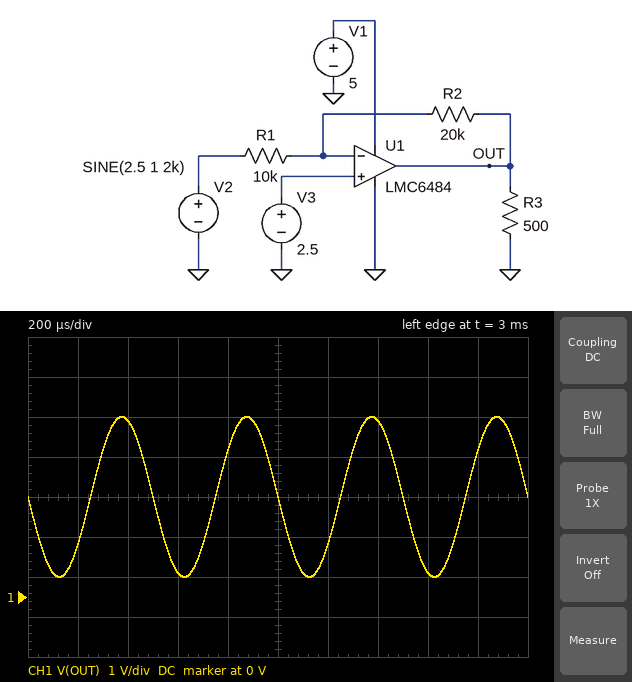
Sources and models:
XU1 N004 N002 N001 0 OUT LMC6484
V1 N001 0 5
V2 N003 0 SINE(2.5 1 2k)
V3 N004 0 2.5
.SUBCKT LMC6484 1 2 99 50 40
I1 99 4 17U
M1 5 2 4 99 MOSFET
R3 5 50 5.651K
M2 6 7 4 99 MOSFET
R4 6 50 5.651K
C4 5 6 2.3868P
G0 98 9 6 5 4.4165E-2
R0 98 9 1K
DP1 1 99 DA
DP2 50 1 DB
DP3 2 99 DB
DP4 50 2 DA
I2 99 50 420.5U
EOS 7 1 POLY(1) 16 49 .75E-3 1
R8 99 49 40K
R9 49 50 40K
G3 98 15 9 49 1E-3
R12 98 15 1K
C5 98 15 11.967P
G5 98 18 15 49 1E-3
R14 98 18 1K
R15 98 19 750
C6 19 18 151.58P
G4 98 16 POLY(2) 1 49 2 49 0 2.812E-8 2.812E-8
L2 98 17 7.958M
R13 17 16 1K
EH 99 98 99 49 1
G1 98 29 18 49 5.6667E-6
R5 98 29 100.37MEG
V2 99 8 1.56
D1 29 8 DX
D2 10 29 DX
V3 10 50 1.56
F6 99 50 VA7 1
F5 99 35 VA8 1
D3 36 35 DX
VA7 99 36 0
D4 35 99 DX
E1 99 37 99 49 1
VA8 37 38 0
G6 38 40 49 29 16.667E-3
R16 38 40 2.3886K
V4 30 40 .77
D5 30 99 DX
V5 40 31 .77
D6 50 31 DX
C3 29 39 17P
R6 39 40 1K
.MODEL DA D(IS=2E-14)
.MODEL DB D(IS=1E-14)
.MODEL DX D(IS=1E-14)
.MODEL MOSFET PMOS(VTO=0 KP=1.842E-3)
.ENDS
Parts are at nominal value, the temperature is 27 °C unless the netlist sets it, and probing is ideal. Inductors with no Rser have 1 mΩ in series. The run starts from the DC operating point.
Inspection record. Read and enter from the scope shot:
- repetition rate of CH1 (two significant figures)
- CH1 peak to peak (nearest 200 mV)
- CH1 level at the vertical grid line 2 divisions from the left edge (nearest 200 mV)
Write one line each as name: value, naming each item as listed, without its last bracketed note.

repetition rate of CH1: 2.0 kHz
CH1 peak to peak: 4.0 V
CH1 level at the vertical grid line 2 divisions from the left edge: 4.4 V
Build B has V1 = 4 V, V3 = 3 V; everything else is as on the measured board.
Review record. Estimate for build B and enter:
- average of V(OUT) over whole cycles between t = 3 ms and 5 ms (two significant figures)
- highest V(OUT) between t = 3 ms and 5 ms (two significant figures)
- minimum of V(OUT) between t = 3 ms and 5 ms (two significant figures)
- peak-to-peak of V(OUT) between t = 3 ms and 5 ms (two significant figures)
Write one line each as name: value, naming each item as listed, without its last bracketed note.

average of V(OUT) over whole cycles between t = 3 ms and 5 ms: 3.3 V
highest V(OUT) between t = 3 ms and 5 ms: 3.9 V
minimum of V(OUT) between t = 3 ms and 5 ms: 2.0 V
peak-to-peak of V(OUT) between t = 3 ms and 5 ms: 1.9 V
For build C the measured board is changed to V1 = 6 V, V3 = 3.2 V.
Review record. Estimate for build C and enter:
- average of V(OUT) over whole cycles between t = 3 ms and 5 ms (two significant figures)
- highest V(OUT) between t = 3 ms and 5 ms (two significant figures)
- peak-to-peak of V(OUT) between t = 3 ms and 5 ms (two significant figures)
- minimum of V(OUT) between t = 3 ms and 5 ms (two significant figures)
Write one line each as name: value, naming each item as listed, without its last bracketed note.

average of V(OUT) over whole cycles between t = 3 ms and 5 ms: 4.5 V
highest V(OUT) between t = 3 ms and 5 ms: 6.0 V
peak-to-peak of V(OUT) between t = 3 ms and 5 ms: 3.4 V
minimum of V(OUT) between t = 3 ms and 5 ms: 2.6 V
